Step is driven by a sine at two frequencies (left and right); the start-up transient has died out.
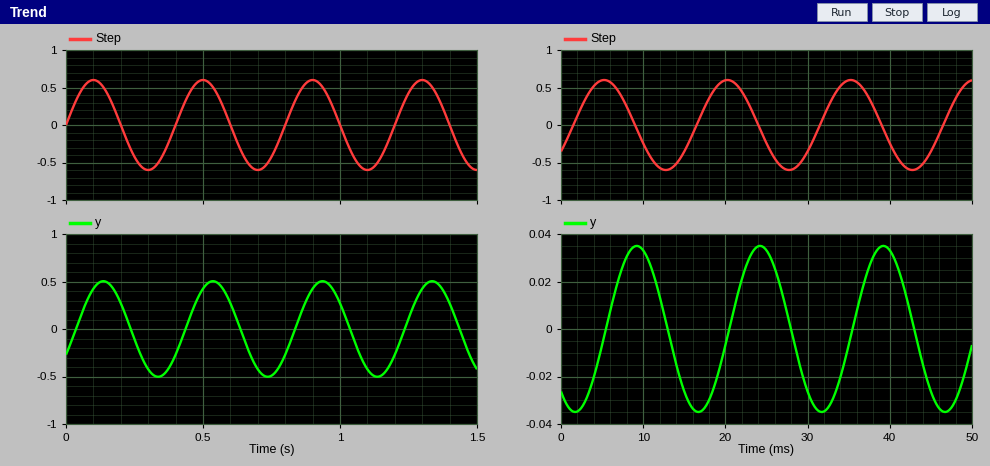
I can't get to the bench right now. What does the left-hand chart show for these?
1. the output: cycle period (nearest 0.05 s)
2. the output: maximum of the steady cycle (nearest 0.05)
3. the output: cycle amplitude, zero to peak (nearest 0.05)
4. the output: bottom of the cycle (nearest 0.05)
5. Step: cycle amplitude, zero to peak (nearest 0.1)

0.40 s
0.50
0.50
-0.50
0.6
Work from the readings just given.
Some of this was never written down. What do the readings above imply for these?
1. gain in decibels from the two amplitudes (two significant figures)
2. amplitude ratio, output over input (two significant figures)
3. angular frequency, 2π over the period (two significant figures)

-1.6 dB
0.83
16 rad/s
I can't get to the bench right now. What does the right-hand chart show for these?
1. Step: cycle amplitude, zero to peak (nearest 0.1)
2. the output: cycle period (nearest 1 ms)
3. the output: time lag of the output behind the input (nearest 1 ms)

0.6
15 ms
4 ms
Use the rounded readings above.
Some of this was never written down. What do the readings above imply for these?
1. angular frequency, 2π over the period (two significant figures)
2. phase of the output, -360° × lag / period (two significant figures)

0.42 rad/ms
-96°
